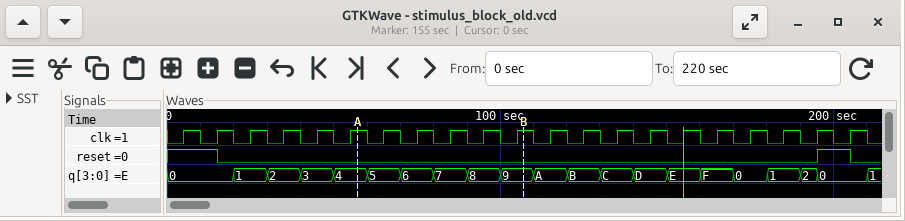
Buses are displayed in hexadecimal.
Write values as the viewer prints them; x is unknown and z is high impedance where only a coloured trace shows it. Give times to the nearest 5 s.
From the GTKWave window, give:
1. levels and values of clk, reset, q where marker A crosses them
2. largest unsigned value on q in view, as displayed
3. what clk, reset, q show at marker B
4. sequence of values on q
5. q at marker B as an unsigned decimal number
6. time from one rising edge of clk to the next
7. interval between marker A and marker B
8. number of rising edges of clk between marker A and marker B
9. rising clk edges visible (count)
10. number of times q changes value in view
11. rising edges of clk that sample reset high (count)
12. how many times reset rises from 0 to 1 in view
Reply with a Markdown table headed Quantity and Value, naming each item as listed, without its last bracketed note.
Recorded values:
| Quantity | Value |
|---|---|
| levels and values of clk, reset, q where marker A crosses them | clk=1, reset=0, q=4 |
| largest unsigned value on q in view, as displayed | F |
| what clk, reset, q show at marker B | clk=1, reset=0, q=9 |
| sequence of values on q | 0, 1, 2, 3, 4, 5, 6, 7, 8, 9, A, B, C, D, E, F, 0, 1, 2, 0, 1 |
| q at marker B as an unsigned decimal number | 9 |
| time from one rising edge of clk to the next | 10 s |
| interval between marker A and marker B | 50 s |
| number of rising edges of clk between marker A and marker B | 5 |
| rising clk edges visible | 21 |
| number of times q changes value in view | 20 |
| rising edges of clk that sample reset high | 3 |
| how many times reset rises from 0 to 1 in view | 1 |
